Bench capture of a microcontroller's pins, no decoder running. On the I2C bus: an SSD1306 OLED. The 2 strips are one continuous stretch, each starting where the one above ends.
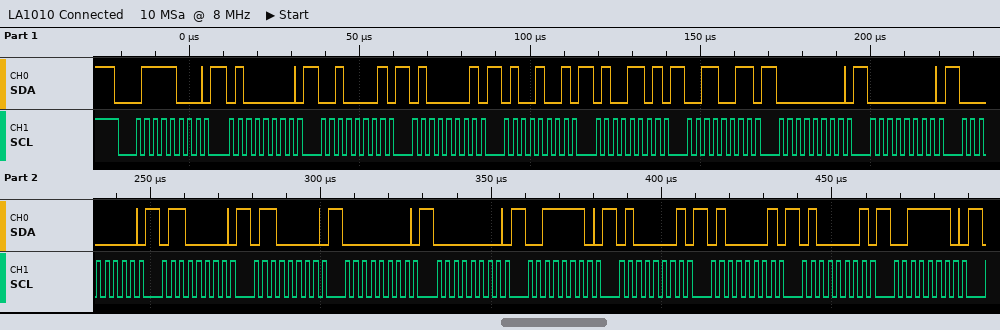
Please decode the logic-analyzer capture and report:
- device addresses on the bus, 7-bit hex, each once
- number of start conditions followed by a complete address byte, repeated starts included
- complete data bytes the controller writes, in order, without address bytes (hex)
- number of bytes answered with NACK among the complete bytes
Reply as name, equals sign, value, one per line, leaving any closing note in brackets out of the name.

device addresses on the bus, 7-bit hex, each once = 0x3C
number of start conditions followed by a complete address byte, repeated starts included = 1
complete data bytes the controller writes, in order, without address bytes = 40 21 41 49 4D 33 00 00 00 60 60 00 00 3E 41 41 41 3E
number of bytes answered with NACK among the complete bytes = 0
